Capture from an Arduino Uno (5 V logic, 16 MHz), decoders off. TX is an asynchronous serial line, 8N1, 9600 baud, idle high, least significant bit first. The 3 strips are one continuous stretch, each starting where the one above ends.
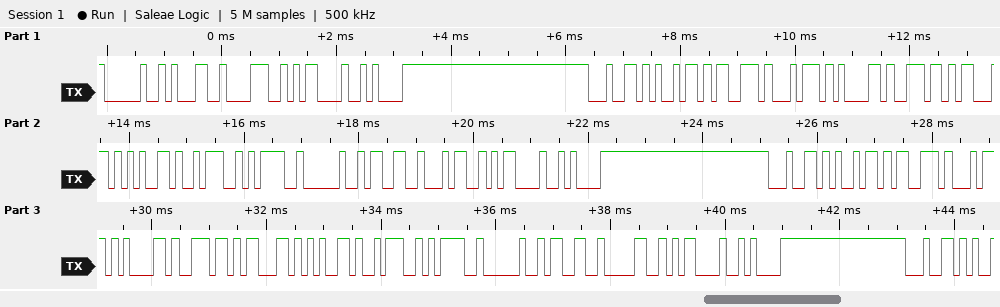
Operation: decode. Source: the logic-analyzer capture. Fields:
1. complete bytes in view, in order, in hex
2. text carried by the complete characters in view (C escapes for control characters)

0x20 0x31 0x38 0x0D 0x0A 0x64 0x69 0x73 0x74 0x61 0x6E 0x63 0x65 0x3A 0x3D 0x20 0x33 0x34 0x0D 0x0A 0x64 0x69 0x73 0x74 0x61 0x6E 0x63 0x65 0x3A 0x3D 0x20 0x33 0x30 0x0D 0x0A 0x64
" 18\r\ndistance:= 34\r\ndistance:= 30\r\nd"
